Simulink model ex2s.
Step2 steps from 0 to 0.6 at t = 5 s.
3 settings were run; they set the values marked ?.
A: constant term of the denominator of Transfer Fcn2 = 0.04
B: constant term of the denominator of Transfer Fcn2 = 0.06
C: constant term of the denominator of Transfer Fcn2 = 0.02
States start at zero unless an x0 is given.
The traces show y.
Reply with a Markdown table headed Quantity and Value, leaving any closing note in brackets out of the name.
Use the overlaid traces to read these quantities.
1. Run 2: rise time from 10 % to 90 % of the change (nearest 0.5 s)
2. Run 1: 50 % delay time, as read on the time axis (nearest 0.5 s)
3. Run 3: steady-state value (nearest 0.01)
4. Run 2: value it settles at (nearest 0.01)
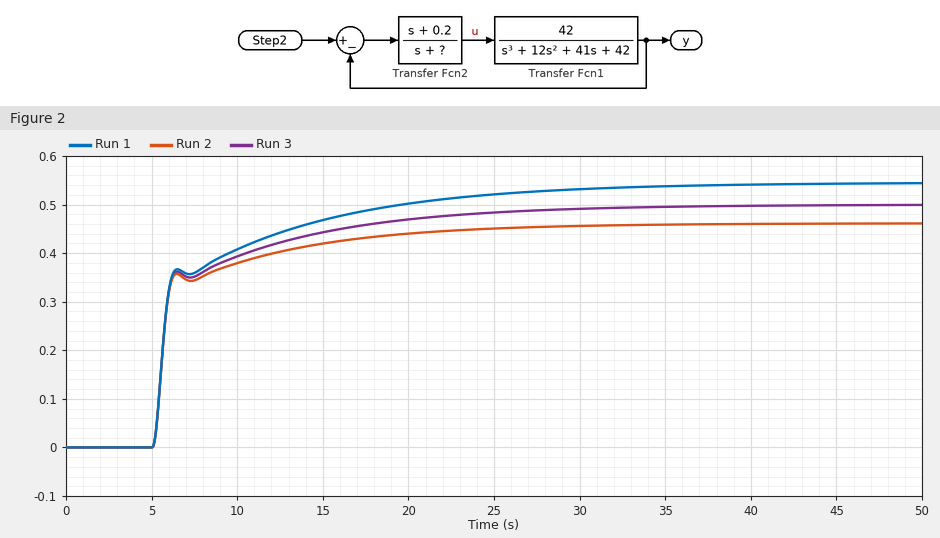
| Quantity | Value |
|---|---|
| Run 2: rise time from 10 % to 90 % of the change | 9.0 s |
| Run 1: 50 % delay time, as read on the time axis | 6.0 s |
| Run 3: steady-state value | 0.50 |
| Run 2: value it settles at | 0.46 |
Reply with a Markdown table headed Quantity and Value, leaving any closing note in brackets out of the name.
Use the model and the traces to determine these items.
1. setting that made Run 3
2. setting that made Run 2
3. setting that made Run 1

| Quantity | Value |
|---|---|
| setting that made Run 3 | A |
| setting that made Run 2 | B |
| setting that made Run 1 | C |
